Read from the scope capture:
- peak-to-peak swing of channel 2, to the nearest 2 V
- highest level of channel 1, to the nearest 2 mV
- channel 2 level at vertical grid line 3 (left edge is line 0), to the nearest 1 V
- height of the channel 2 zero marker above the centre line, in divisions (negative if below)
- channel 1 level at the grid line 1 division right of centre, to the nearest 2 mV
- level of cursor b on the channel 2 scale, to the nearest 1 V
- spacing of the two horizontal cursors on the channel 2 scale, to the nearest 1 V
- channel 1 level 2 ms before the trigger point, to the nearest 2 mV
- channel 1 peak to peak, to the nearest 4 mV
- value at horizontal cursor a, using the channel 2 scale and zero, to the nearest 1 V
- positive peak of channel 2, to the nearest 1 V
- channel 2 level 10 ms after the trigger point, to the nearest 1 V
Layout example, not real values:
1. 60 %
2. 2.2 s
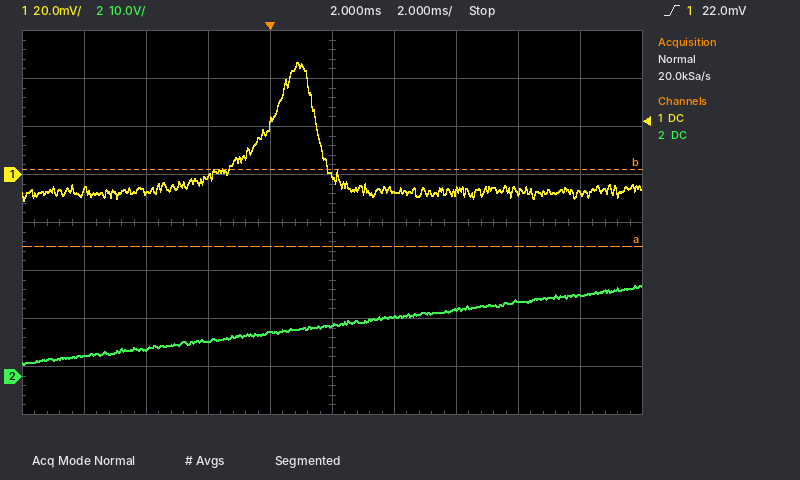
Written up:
1. 16 V
2. 46 mV
3. 7 V
4. -3.2 div
5. -8 mV
6. 43 V
7. 16 V
8. 0 mV
9. 56 mV
10. 27 V
11. 19 V
12. 17 V
